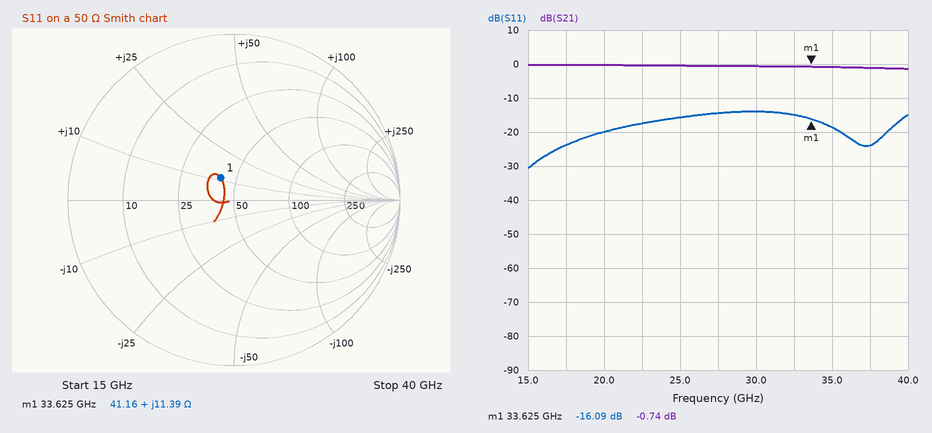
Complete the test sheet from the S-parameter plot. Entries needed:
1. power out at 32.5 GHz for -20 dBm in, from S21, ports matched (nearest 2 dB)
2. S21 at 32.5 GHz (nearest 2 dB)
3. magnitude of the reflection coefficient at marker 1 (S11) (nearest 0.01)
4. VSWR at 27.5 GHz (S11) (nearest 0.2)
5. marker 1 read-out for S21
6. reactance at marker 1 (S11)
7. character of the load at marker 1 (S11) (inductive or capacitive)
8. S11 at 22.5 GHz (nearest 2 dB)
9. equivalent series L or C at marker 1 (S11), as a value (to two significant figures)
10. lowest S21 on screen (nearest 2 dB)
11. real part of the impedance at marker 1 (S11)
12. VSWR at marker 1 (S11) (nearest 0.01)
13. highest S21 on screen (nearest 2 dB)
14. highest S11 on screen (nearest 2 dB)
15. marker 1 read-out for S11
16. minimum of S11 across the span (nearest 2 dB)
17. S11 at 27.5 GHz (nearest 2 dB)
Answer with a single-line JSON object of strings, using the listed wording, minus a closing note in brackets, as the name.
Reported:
{"power out at 32.5 GHz for -20 dBm in, from S21, ports matched": "-20 dBm", "S21 at 32.5 GHz": "0 dB", "magnitude of the reflection coefficient at marker 1 (S11)": "0.16", "VSWR at 27.5 GHz (S11)": "1.4", "marker 1 read-out for S21": "-0.74 dB", "reactance at marker 1": "+11.39 Ω", "character of the load at marker 1 (S11)": "inductive", "S11 at 22.5 GHz": "-18 dB", "equivalent series L or C at marker 1 (S11), as a value": "54 pH", "lowest S21 on screen": "-2 dB", "real part of the impedance at marker 1": "41.16 Ω", "VSWR at marker 1 (S11)": "1.37", "highest S21 on screen": "0 dB", "highest S11 on screen": "-14 dB", "marker 1 read-out for S11": "-16.09 dB", "minimum of S11 across the span": "-30 dB", "S11 at 27.5 GHz": "-14 dB"}
